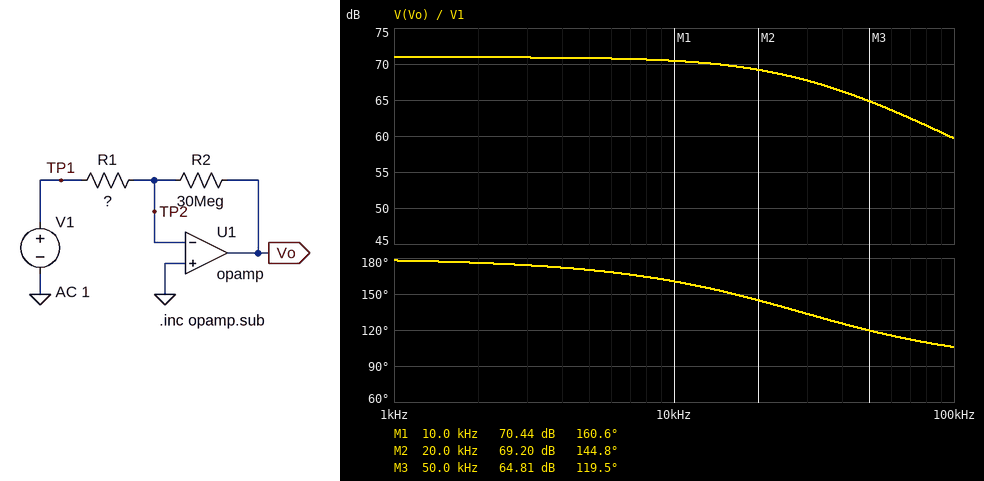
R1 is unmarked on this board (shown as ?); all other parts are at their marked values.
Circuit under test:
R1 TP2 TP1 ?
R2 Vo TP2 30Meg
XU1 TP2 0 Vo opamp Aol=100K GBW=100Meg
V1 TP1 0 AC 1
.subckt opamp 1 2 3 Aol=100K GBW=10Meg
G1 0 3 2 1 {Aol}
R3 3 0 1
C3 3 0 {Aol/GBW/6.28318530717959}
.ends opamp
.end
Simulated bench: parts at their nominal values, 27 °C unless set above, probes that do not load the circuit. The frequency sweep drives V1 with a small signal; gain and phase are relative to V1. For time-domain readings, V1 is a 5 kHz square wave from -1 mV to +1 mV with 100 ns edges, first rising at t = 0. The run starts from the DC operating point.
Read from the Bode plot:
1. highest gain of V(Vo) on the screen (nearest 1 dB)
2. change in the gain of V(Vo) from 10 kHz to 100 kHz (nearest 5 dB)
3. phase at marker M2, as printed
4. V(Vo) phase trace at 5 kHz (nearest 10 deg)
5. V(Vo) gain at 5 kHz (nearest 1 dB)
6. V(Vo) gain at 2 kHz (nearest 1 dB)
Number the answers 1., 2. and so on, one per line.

1. 71 dB
2. -10 dB
3. 144.8 deg
4. 170 deg
5. 71 dB
6. 71 dB
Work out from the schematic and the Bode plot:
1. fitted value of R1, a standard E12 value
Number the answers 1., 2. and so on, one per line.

1. 8.2 kΩ
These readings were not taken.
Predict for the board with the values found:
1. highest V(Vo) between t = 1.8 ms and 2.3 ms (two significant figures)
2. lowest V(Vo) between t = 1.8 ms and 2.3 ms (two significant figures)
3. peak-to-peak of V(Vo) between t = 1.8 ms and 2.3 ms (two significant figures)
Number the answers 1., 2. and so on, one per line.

1. 3.5 V
2. -3.5 V
3. 7.1 V
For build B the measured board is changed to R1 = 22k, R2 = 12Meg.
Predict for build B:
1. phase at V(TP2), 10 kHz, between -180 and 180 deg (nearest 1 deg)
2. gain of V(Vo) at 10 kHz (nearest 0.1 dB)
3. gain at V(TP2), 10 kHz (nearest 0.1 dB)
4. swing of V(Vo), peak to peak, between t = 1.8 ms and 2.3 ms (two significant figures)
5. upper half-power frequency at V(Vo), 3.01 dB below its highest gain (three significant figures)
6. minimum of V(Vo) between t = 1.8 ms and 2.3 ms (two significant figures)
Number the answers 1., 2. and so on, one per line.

1. 81 deg
2. 54.7 dB
3. -25.3 dB
4. 1.1 V
5. 184 kHz
6. -540 mV
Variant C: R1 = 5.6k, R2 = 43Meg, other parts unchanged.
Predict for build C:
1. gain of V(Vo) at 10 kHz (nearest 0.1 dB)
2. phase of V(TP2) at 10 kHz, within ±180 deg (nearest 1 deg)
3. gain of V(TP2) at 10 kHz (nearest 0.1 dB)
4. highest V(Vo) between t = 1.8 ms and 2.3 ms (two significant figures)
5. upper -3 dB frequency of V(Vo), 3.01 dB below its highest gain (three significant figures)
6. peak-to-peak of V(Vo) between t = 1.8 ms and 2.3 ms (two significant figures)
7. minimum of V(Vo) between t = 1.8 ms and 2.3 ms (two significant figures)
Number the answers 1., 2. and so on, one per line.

1. 75.3 dB
2. 49 deg
3. -4.7 dB
4. 7.1 V
5. 14.0 kHz
6. 14 V
7. -7.1 V
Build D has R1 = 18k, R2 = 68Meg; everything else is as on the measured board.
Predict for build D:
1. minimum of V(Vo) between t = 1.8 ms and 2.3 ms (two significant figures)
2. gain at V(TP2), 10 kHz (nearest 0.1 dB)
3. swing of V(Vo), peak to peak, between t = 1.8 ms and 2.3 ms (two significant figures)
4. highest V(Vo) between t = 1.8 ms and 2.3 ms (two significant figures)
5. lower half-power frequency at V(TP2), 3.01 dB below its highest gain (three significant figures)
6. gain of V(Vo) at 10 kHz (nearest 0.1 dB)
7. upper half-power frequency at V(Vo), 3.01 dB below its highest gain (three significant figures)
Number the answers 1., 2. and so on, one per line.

1. -3.6 V
2. -9.3 dB
3. 7.3 V
4. 3.6 V
5. 27.4 kHz
6. 70.7 dB
7. 27.5 kHz
